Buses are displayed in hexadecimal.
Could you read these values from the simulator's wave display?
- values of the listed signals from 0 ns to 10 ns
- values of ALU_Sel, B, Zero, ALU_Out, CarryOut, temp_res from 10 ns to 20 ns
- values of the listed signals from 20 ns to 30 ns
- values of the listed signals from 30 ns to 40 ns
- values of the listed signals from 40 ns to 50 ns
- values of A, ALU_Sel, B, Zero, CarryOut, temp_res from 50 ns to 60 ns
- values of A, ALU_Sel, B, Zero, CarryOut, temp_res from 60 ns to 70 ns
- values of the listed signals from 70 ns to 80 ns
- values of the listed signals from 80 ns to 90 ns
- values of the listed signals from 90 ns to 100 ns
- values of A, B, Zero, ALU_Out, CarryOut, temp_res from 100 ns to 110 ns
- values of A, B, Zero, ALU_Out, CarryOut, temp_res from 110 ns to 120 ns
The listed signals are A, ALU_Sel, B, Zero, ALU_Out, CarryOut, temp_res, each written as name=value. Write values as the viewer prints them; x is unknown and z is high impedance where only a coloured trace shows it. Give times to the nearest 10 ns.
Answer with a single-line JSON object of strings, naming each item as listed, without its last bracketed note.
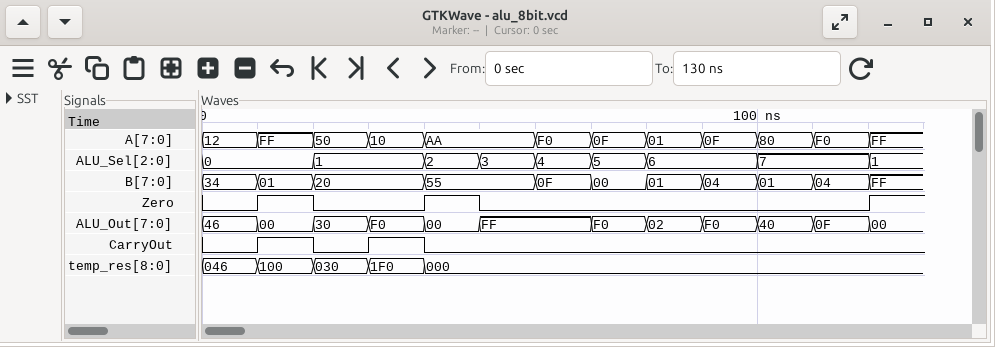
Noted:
{"values of the listed signals from 0 ns to 10 ns": "A=12, ALU_Sel=0, B=34, Zero=0, ALU_Out=46, CarryOut=0, temp_res=046", "values of ALU_Sel, B, Zero, ALU_Out, CarryOut, temp_res from 10 ns to 20 ns": "ALU_Sel=0, B=01, Zero=1, ALU_Out=00, CarryOut=1, temp_res=100", "values of the listed signals from 20 ns to 30 ns": "A=50, ALU_Sel=1, B=20, Zero=0, ALU_Out=30, CarryOut=0, temp_res=030", "values of the listed signals from 30 ns to 40 ns": "A=10, ALU_Sel=1, B=20, Zero=0, ALU_Out=F0, CarryOut=1, temp_res=1F0", "values of the listed signals from 40 ns to 50 ns": "A=AA, ALU_Sel=2, B=55, Zero=1, ALU_Out=00, CarryOut=0, temp_res=000", "values of A, ALU_Sel, B, Zero, CarryOut, temp_res from 50 ns to 60 ns": "A=AA, ALU_Sel=3, B=55, Zero=0, CarryOut=0, temp_res=000", "values of A, ALU_Sel, B, Zero, CarryOut, temp_res from 60 ns to 70 ns": "A=F0, ALU_Sel=4, B=0F, Zero=0, CarryOut=0, temp_res=000", "values of the listed signals from 70 ns to 80 ns": "A=0F, ALU_Sel=5, B=00, Zero=0, ALU_Out=F0, CarryOut=0, temp_res=000", "values of the listed signals from 80 ns to 90 ns": "A=01, ALU_Sel=6, B=01, Zero=0, ALU_Out=02, CarryOut=0, temp_res=000", "values of the listed signals from 90 ns to 100 ns": "A=0F, ALU_Sel=6, B=04, Zero=0, ALU_Out=F0, CarryOut=0, temp_res=000", "values of A, B, Zero, ALU_Out, CarryOut, temp_res from 100 ns to 110 ns": "A=80, B=01, Zero=0, ALU_Out=40, CarryOut=0, temp_res=000", "values of A, B, Zero, ALU_Out, CarryOut, temp_res from 110 ns to 120 ns": "A=F0, B=04, Zero=0, ALU_Out=0F, CarryOut=0, temp_res=000"}
